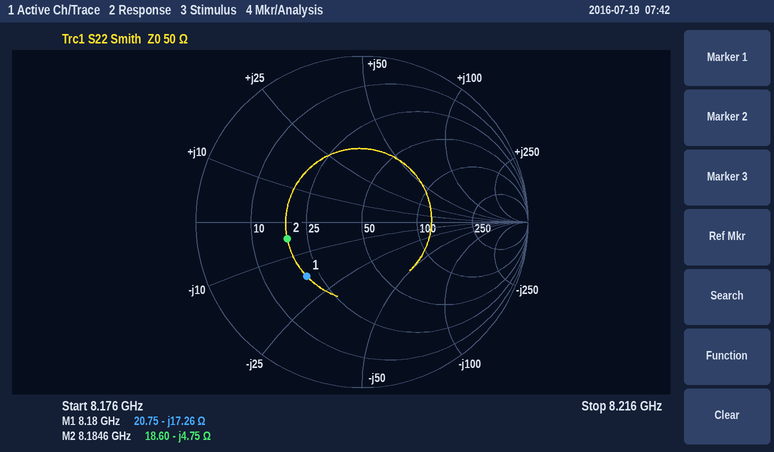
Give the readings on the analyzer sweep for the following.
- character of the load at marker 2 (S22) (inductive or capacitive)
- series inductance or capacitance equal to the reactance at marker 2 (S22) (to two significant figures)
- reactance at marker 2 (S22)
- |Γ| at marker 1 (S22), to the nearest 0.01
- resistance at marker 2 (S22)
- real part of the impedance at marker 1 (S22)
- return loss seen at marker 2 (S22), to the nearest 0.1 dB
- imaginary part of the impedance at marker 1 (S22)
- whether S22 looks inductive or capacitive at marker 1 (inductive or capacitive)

capacitive
4.1 pF
-4.75 Ω
0.47
18.60 Ω
20.75 Ω
6.7 dB
-17.26 Ω
capacitive
